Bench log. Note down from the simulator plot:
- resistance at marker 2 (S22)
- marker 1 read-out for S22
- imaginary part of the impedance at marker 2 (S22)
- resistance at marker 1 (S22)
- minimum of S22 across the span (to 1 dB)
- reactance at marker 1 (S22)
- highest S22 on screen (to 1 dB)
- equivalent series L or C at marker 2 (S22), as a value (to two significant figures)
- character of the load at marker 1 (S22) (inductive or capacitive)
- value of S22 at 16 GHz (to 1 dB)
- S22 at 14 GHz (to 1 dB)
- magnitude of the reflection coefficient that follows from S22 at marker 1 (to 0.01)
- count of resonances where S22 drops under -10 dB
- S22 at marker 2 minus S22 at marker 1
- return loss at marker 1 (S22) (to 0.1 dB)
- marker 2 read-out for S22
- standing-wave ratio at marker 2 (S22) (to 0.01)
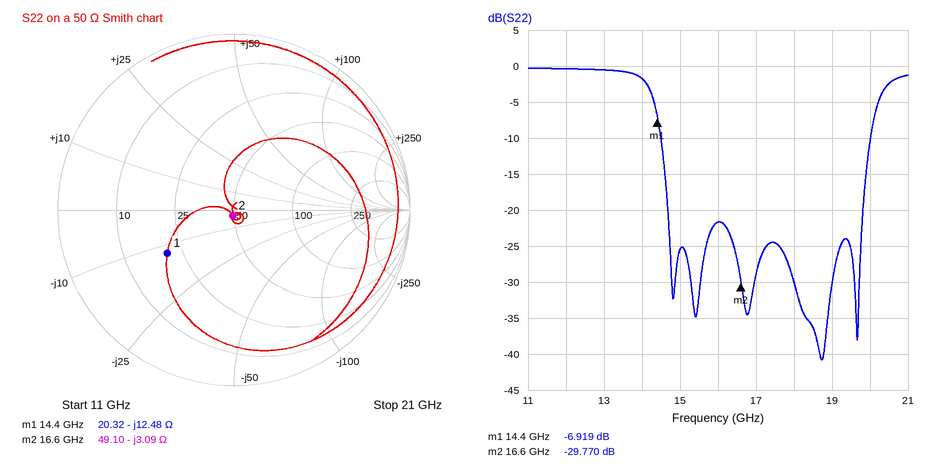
49.10 Ω
-6.919 dB
-3.09 Ω
20.32 Ω
-41 dB
-12.48 Ω
0 dB
3.1 pF
capacitive
-22 dB
-2 dB
0.45
5
-22.851 dB
6.9 dB
-29.770 dB
1.07
